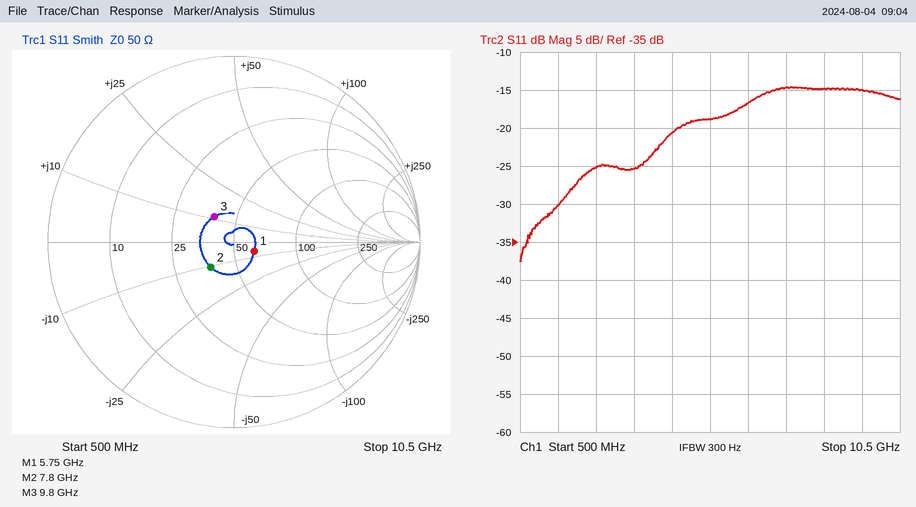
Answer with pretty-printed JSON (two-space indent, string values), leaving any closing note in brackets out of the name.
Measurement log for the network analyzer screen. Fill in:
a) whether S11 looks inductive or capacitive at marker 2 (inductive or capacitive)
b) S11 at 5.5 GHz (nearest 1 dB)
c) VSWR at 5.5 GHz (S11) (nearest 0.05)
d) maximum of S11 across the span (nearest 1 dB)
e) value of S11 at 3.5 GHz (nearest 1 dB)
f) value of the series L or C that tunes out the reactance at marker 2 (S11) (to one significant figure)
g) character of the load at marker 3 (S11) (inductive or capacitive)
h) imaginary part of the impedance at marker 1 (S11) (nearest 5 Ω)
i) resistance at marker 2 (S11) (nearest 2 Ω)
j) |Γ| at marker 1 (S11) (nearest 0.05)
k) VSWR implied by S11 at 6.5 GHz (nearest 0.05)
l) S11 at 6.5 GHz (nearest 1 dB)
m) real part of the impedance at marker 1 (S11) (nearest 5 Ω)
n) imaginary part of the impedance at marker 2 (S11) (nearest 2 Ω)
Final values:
{
  "whether S11 looks inductive or capacitive at marker 2": "capacitive",
  "S11 at 5.5 GHz": "-19 dB",
  "VSWR at 5.5 GHz (S11)": "1.25",
  "maximum of S11 across the span": "-15 dB",
  "value of S11 at 3.5 GHz": "-25 dB",
  "value of the series L or C that tunes out the reactance at marker 2 (S11)": "200 pH",
  "character of the load at marker 3 (S11)": "inductive",
  "imaginary part of the impedance at marker 1 (S11)": "-5 Ω",
  "resistance at marker 2 (S11)": "38 Ω",
  "|Γ| at marker 1 (S11)": "0.10",
  "VSWR implied by S11 at 6.5 GHz": "1.35",
  "S11 at 6.5 GHz": "-17 dB",
  "real part of the impedance at marker 1 (S11)": "60 Ω",
  "imaginary part of the impedance at marker 2 (S11)": "-10 Ω"
}
